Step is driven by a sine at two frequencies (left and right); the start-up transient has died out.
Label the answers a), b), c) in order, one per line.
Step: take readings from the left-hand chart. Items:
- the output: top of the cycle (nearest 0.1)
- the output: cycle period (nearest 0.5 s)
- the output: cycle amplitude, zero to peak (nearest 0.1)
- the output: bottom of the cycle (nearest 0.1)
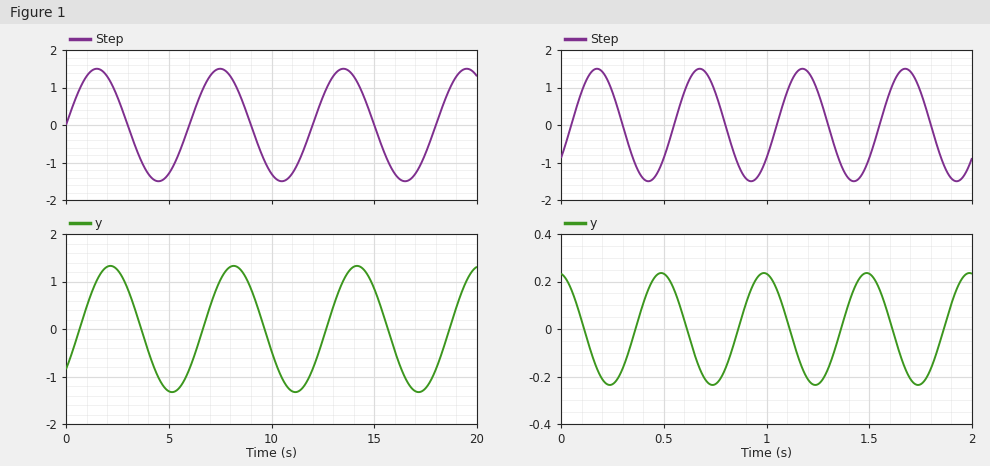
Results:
a) 1.3
b) 6.0 s
c) 1.3
d) -1.3
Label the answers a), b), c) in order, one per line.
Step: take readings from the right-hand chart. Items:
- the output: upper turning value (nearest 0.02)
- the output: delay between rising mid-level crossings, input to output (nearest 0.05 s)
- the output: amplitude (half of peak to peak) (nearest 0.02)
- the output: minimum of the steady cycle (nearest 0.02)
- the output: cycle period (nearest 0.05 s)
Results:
a) 0.24
b) 0.30 s
c) 0.24
d) -0.24
e) 0.50 s
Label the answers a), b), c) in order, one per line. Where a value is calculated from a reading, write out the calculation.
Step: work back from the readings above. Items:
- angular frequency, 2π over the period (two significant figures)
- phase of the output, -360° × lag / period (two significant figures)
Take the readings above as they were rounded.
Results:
a) 2π / 0.5 = 13 rad/s
b) -360 × 0.3 / 0.5 = -220°
